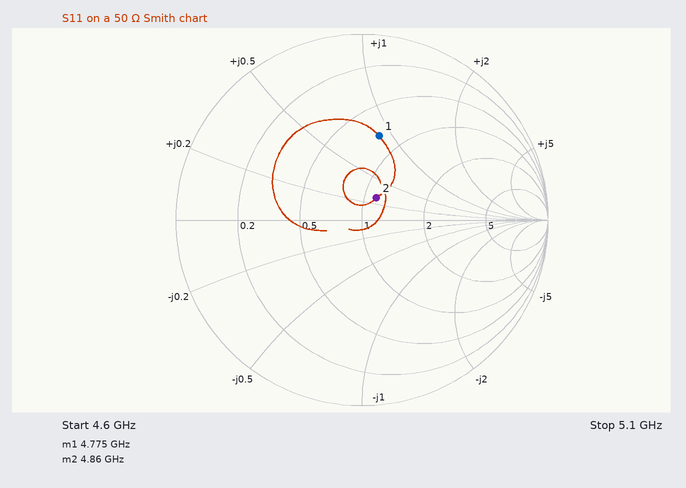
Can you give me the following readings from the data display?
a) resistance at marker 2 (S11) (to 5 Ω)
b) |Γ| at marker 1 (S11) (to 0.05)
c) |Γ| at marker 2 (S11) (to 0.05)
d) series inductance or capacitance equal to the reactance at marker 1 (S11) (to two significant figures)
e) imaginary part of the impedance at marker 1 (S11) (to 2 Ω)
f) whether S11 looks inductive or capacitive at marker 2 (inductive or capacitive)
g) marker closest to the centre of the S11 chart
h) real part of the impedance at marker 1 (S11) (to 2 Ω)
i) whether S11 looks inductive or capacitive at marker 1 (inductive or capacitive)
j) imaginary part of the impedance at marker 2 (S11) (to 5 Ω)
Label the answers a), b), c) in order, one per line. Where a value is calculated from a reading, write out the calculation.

a) 55 Ω
b) 0.45
c) 0.15
d) L = 44 Ω/(2π × 4.775 GHz) ≈ 1.5 nH
e) +44 Ω
f) inductive
g) marker 2
h) 38 Ω
i) inductive
j) +15 Ω
